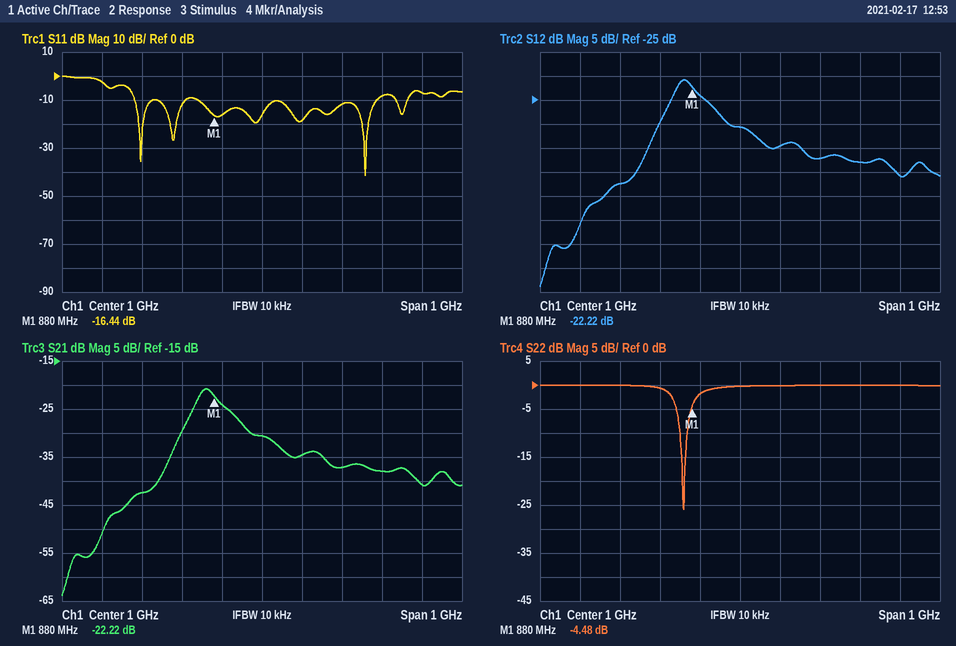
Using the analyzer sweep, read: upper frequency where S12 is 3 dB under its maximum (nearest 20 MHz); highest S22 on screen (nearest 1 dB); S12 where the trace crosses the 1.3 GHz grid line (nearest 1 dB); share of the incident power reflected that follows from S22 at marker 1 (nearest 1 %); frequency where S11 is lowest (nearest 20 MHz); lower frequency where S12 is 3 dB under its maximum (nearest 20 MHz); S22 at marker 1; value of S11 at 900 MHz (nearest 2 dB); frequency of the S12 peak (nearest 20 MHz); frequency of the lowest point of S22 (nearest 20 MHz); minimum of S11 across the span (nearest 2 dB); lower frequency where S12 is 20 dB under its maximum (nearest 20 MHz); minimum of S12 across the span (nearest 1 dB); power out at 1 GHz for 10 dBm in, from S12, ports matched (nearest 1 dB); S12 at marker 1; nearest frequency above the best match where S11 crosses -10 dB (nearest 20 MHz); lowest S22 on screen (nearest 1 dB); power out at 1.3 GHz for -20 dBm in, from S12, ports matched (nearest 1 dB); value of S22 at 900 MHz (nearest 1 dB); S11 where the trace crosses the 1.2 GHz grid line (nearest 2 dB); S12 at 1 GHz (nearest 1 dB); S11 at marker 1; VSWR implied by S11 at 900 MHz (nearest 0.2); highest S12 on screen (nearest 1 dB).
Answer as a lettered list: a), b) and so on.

a) 900 MHz
b) 0 dB
c) -38 dB
d) 36 %
e) 1.26 GHz
f) 840 MHz
g) -4.48 dB
h) -16 dB
i) 860 MHz
j) 860 MHz
k) -42 dB
l) 740 MHz
m) -64 dB
n) -21 dBm
o) -22.22 dB
p) 1.28 GHz
q) -26 dB
r) -58 dBm
s) -2 dB
t) -12 dB
u) -31 dB
v) -16.44 dB
w) 1.4
x) -21 dB
